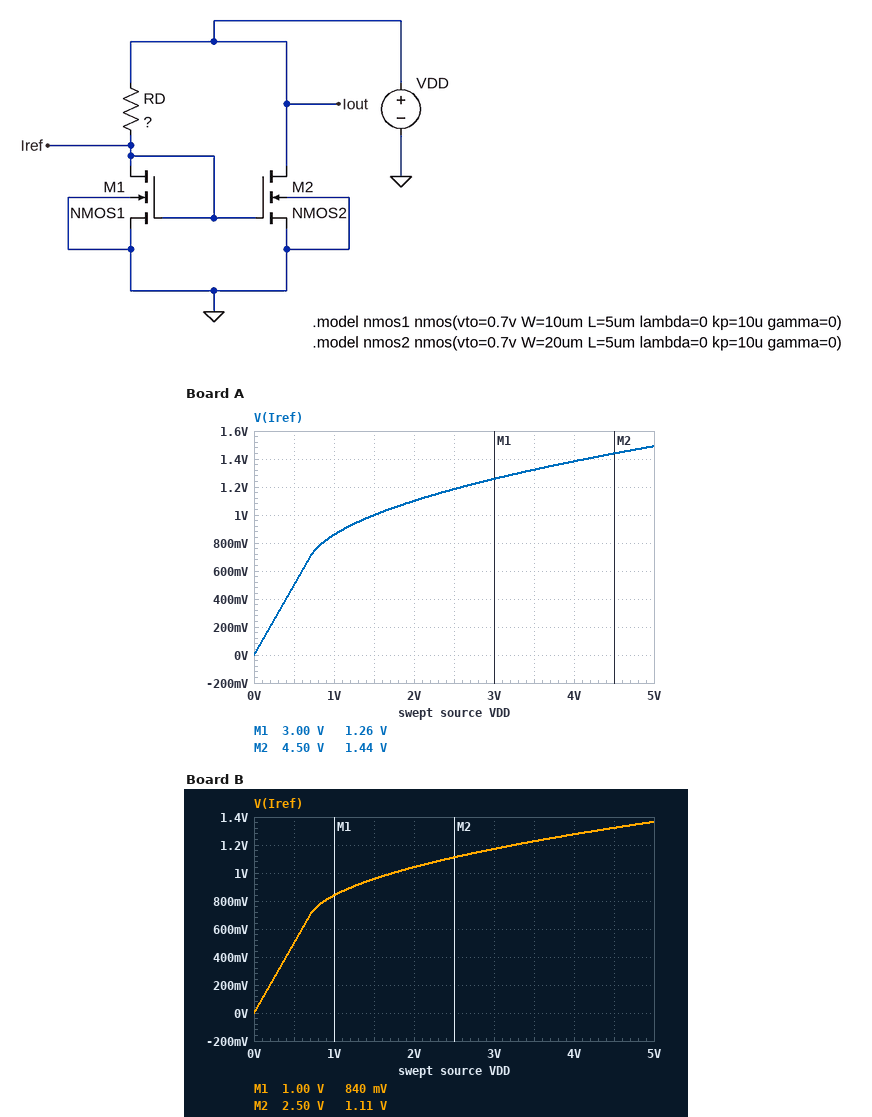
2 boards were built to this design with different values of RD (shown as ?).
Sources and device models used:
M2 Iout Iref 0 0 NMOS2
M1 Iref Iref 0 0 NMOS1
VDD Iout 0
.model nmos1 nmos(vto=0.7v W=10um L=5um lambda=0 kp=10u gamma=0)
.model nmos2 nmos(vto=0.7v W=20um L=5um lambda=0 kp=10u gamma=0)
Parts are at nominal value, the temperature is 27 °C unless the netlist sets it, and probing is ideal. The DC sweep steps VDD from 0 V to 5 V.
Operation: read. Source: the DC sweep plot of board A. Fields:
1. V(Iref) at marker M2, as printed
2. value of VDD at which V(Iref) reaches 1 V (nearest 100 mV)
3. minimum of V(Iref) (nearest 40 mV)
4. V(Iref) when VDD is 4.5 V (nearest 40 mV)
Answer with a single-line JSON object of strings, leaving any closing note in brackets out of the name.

{"V(Iref) at marker M2, as printed": "1.44 V", "value of VDD at which V(Iref) reaches 1 V": "1.5 V", "minimum of V(Iref)": "0 V", "V(Iref) when VDD is 4.5 V": "1.44 V"}
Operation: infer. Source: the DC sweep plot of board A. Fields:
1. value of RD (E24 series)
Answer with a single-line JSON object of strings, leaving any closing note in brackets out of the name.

{"value of RD": "560 kΩ"}
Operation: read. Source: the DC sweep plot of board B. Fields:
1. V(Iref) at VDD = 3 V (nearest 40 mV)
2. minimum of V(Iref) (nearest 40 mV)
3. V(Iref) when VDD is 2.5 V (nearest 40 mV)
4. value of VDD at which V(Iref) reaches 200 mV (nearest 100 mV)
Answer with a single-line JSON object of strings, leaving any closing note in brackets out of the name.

{"V(Iref) at VDD = 3 V": "1.16 V", "minimum of V(Iref)": "0 V", "V(Iref) when VDD is 2.5 V": "1.12 V", "value of VDD at which V(Iref) reaches 200 mV": "200 mV"}
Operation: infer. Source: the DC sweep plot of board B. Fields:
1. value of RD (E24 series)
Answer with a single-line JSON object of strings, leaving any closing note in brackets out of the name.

{"value of RD": "820 kΩ"}
